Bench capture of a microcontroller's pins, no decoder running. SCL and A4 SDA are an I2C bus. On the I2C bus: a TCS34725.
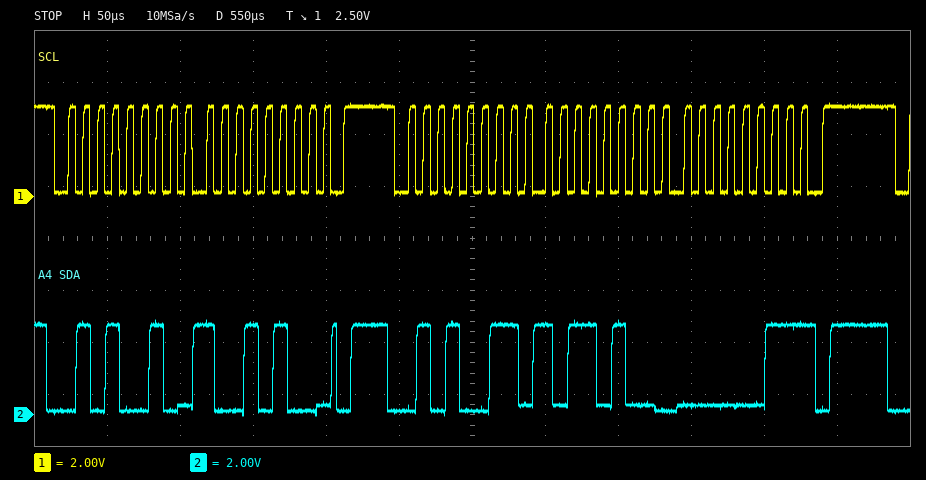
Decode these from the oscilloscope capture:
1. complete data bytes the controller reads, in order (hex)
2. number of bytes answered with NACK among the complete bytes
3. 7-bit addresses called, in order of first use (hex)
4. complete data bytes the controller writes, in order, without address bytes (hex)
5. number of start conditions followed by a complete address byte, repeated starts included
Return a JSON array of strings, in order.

["B4 03", "1", "0x29", "94", "2"]
